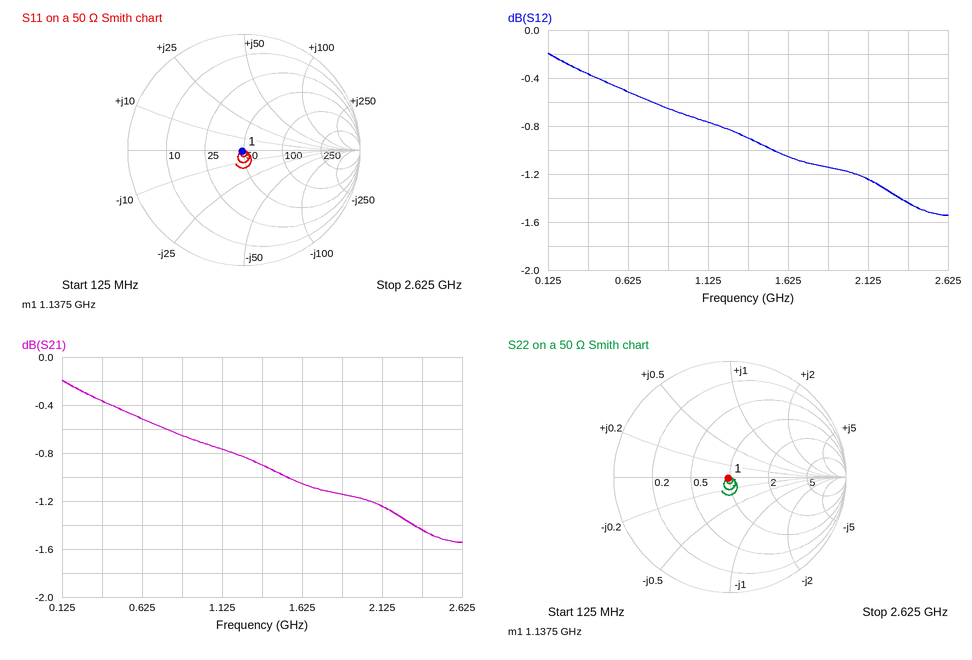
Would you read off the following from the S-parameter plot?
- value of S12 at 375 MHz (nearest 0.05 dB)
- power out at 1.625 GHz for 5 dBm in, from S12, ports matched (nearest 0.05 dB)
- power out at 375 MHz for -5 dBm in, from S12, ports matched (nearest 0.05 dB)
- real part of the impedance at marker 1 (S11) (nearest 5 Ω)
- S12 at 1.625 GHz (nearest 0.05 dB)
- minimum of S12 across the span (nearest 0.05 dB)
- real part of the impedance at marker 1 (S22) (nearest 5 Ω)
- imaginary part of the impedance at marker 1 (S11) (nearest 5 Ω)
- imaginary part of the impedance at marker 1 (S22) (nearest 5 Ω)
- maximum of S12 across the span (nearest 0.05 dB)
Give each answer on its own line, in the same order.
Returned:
-0.35 dB
3.95 dBm
-5.35 dBm
50 Ω
-1.05 dB
-1.55 dB
50 Ω
0 Ω
0 Ω
-0.20 dB
